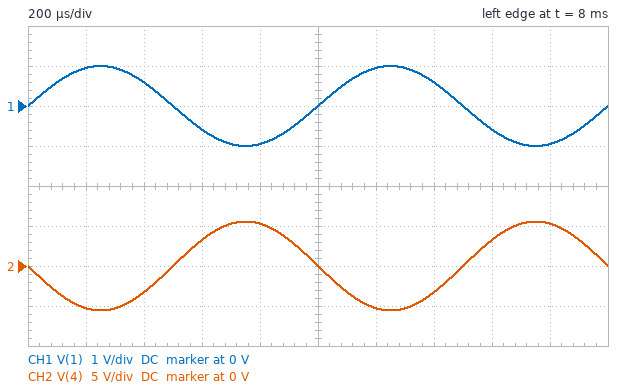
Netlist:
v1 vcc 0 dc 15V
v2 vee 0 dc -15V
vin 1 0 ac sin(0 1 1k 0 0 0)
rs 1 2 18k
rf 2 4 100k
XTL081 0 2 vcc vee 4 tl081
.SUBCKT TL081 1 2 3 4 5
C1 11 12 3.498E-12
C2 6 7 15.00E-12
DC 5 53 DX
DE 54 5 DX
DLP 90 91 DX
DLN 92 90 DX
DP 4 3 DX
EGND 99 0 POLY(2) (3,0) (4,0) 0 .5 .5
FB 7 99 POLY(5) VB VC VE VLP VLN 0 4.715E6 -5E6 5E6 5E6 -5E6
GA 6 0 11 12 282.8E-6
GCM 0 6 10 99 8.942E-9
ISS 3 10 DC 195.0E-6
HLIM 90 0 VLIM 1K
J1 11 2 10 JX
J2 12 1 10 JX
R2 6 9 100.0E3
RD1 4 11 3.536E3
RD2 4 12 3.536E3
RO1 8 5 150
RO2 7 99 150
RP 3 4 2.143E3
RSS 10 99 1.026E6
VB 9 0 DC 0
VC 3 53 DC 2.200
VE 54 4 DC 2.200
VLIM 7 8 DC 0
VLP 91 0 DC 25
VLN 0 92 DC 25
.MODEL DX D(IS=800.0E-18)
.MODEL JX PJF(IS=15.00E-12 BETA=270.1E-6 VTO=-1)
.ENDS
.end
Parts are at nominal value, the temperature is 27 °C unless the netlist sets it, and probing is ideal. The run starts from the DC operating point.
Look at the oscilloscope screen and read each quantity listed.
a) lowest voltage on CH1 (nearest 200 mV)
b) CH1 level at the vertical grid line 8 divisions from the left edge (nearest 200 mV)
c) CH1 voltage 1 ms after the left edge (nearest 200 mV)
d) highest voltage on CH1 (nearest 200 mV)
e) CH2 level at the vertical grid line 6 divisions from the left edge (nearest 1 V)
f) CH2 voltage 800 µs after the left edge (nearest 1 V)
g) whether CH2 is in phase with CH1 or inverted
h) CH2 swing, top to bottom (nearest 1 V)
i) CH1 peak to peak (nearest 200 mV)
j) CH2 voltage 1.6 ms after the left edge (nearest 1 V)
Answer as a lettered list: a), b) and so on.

a) -1.0 V
b) -600 mV
c) 0 V
d) 1.0 V
e) -5 V
f) 5 V
g) inverted
h) 11 V
i) 2.0 V
j) 3 V
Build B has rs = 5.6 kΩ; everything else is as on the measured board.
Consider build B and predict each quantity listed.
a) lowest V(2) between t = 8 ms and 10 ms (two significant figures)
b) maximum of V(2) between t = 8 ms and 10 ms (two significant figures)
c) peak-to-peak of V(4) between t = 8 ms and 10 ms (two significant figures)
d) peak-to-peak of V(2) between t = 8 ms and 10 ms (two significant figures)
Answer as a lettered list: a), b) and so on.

a) -230 mV
b) 230 mV
c) 27 V
d) 470 mV
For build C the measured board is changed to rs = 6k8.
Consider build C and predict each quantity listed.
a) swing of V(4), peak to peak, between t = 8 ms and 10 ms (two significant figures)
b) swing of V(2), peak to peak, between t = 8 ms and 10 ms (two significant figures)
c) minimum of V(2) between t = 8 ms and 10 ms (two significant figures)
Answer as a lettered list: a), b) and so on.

a) 27 V
b) 160 mV
c) -82 mV
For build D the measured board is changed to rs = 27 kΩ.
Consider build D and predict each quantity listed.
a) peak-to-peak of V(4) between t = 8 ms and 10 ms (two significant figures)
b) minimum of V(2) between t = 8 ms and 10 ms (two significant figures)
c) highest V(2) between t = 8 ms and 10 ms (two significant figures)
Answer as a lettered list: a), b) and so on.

a) 7.4 V
b) -1.1 mV
c) 1.1 mV
